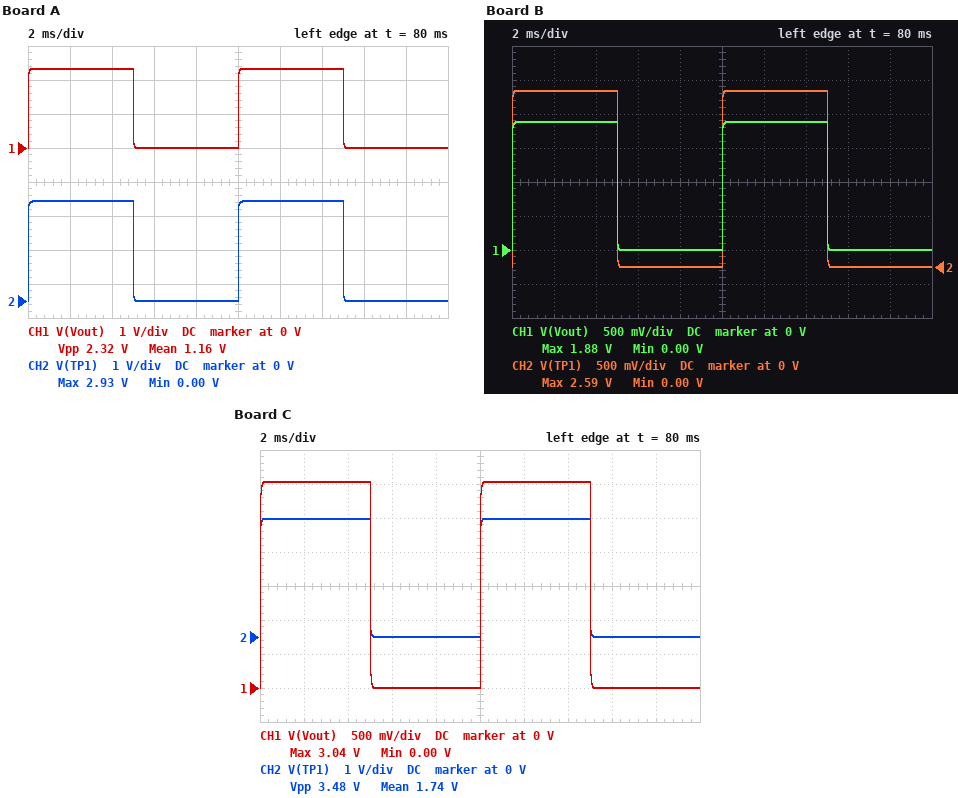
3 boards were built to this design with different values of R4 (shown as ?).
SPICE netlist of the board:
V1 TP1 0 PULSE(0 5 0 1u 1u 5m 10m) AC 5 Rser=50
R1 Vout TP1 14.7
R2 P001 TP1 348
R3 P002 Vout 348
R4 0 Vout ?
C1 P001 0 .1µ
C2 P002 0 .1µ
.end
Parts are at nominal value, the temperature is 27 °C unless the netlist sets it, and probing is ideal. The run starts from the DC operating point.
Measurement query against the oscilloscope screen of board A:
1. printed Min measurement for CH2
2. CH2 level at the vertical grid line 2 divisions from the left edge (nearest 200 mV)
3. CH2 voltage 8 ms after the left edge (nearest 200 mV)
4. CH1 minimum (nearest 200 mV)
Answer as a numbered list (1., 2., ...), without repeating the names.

1. 0.00 V
2. 3.0 V
3. 0 V
4. 0 V
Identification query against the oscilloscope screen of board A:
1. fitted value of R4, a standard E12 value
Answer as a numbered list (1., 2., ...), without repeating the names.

1. 56 Ω
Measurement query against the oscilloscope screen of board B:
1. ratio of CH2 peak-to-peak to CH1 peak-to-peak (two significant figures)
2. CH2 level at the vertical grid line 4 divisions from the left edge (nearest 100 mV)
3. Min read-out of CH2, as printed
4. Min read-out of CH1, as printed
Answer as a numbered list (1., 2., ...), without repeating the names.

1. 1.4
2. 0 V
3. 0.00 V
4. 0.00 V
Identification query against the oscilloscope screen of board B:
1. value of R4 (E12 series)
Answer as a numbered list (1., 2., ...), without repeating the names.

1. 39 Ω
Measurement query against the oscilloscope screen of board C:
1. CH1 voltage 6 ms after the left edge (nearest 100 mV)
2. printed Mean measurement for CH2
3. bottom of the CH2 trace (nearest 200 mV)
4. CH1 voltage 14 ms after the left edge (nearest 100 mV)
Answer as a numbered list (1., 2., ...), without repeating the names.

1. 0 V
2. 1.74 V
3. 0 V
4. 3.0 V
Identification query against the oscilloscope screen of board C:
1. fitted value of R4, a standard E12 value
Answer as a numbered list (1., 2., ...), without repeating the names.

1. 100 Ω
